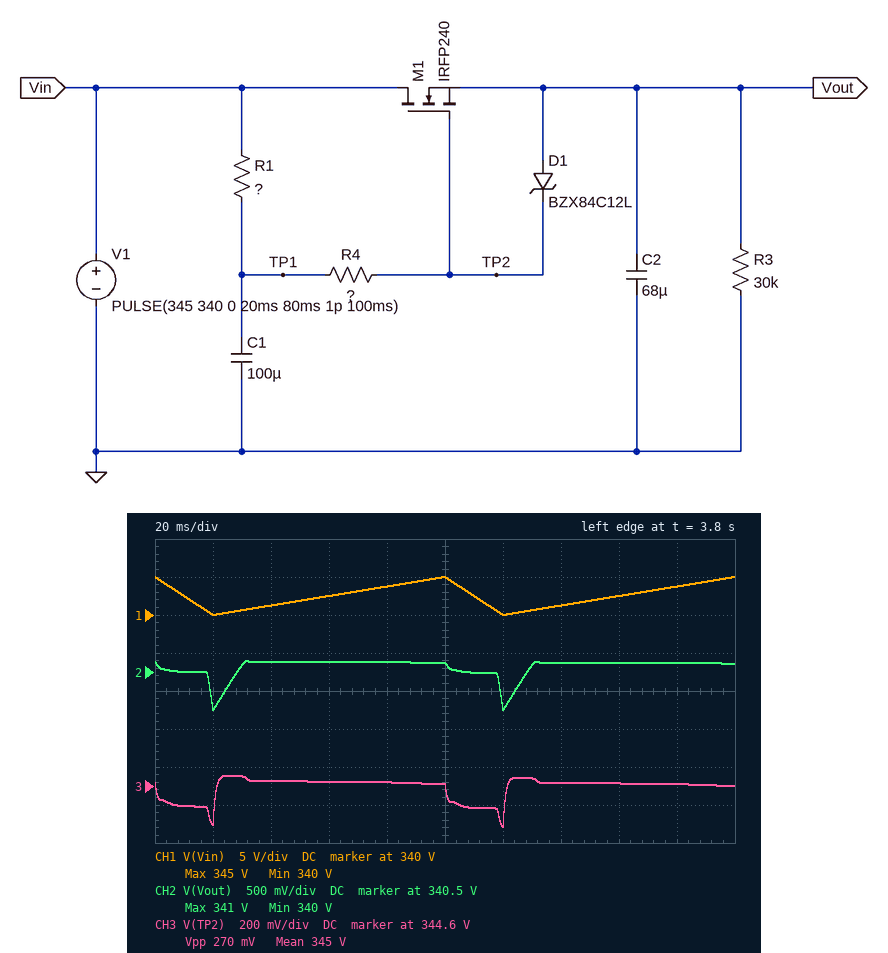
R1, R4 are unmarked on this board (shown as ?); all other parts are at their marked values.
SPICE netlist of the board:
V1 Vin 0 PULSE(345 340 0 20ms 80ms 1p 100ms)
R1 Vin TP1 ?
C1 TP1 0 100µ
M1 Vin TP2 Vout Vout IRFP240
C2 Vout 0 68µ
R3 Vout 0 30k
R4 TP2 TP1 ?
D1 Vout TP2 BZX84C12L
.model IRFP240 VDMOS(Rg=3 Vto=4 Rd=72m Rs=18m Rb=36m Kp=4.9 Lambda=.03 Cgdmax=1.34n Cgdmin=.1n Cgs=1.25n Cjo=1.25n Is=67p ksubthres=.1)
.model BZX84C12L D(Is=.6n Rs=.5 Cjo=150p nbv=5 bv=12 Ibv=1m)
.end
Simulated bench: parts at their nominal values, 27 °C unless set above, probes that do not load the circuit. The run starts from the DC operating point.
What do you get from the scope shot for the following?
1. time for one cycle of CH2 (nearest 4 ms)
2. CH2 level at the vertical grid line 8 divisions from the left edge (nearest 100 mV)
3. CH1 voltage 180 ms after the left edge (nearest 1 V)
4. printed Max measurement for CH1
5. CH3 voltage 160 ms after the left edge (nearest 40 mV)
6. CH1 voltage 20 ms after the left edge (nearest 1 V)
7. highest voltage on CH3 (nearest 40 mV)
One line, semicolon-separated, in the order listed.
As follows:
100 ms; 340.6 V; 344 V; 345 V; 344.60 V; 340 V; 344.64 V
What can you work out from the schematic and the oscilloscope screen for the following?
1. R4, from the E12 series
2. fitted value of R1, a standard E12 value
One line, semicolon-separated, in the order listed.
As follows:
330 kΩ; 220 kΩ
